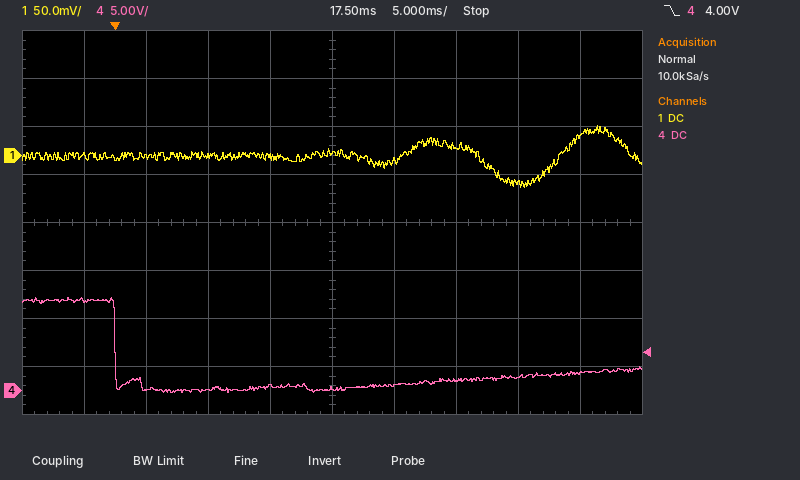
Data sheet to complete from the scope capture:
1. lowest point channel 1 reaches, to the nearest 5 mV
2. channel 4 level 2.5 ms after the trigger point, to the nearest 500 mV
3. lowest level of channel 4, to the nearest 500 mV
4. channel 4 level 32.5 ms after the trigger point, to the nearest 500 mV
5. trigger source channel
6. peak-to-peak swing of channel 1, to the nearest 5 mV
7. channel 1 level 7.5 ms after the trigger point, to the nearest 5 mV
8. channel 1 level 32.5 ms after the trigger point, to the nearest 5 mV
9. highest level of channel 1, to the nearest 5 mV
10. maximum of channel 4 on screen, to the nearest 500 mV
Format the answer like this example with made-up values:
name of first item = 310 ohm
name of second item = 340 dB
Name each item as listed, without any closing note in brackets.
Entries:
lowest point channel 1 reaches, to the nearest 5 mV = -35 mV
channel 4 level 2.5 ms after the trigger point, to the nearest 500 mV = 0.0 V
lowest level of channel 4, to the nearest 500 mV = 0.0 V
channel 4 level 32.5 ms after the trigger point, to the nearest 500 mV = 1.5 V
trigger source channel = channel 4
peak-to-peak swing of channel 1, to the nearest 5 mV = 65 mV
channel 1 level 7.5 ms after the trigger point, to the nearest 5 mV = 0 mV
channel 1 level 32.5 ms after the trigger point, to the nearest 5 mV = -30 mV
highest level of channel 1, to the nearest 5 mV = 30 mV
maximum of channel 4 on screen, to the nearest 500 mV = 9.5 V
